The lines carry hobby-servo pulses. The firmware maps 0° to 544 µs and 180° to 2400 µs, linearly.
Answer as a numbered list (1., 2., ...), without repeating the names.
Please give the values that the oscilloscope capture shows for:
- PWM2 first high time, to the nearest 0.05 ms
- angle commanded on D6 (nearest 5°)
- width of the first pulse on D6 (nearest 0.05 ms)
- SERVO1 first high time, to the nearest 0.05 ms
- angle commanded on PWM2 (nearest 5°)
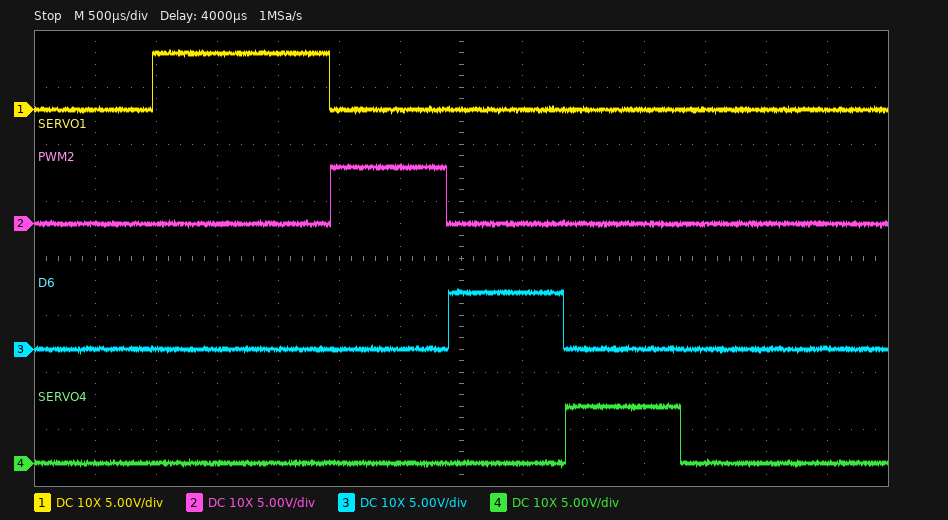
1. 0.95 ms
2. 40°
3. 0.95 ms
4. 1.45 ms
5. 40°
